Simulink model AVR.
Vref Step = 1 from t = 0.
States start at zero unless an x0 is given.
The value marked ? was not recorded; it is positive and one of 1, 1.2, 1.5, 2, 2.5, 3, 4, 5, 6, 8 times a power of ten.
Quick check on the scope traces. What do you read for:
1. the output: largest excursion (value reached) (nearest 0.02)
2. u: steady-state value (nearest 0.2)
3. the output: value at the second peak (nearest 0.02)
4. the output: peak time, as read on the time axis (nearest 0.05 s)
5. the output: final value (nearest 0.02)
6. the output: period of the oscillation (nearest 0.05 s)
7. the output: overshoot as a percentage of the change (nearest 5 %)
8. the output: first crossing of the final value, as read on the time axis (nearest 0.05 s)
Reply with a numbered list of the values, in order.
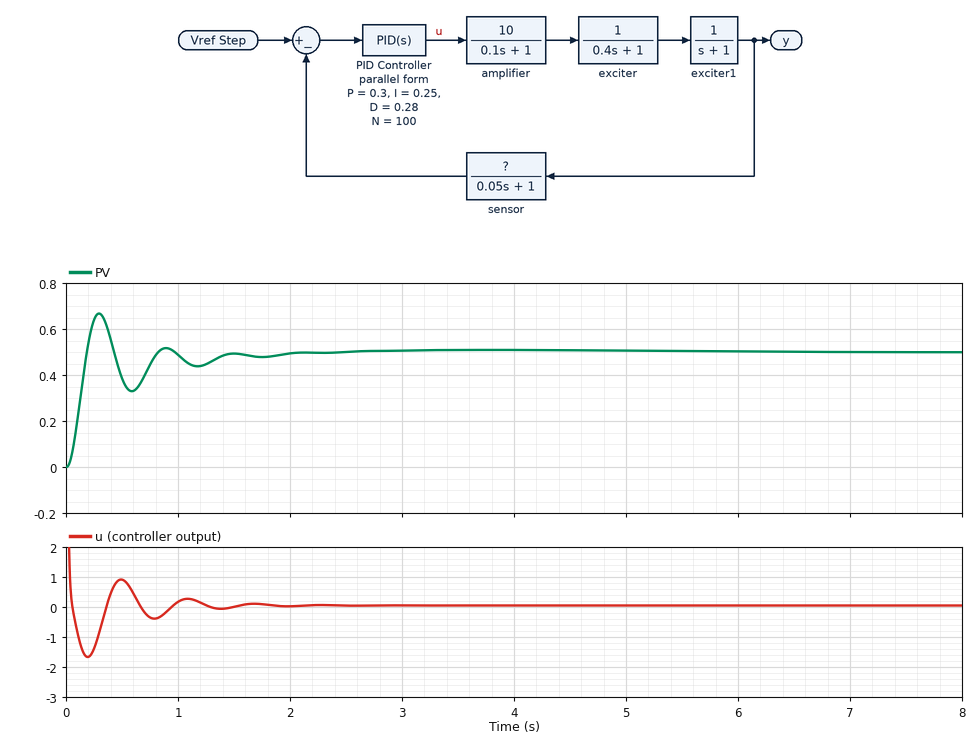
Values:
1. 0.66
2. 0.0
3. 0.52
4. 0.30 s
5. 0.50
6. 0.60 s
7. 35 %
8. 0.20 s
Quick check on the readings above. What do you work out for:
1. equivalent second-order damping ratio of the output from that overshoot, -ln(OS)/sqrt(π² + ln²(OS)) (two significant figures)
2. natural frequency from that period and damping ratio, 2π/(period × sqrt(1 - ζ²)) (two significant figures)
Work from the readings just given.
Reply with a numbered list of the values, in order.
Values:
1. 0.32
2. 11 rad/s
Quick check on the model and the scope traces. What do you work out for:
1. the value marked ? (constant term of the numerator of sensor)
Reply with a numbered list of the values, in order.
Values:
1. 2
